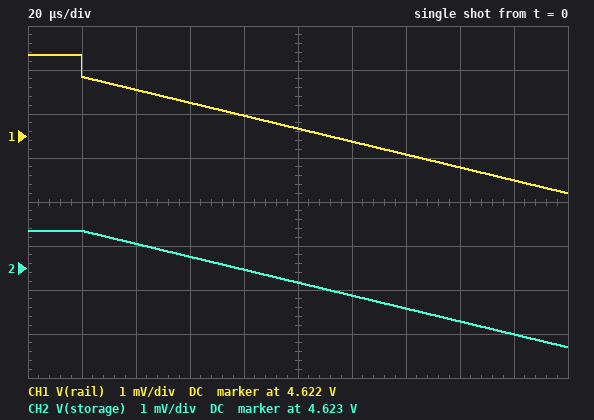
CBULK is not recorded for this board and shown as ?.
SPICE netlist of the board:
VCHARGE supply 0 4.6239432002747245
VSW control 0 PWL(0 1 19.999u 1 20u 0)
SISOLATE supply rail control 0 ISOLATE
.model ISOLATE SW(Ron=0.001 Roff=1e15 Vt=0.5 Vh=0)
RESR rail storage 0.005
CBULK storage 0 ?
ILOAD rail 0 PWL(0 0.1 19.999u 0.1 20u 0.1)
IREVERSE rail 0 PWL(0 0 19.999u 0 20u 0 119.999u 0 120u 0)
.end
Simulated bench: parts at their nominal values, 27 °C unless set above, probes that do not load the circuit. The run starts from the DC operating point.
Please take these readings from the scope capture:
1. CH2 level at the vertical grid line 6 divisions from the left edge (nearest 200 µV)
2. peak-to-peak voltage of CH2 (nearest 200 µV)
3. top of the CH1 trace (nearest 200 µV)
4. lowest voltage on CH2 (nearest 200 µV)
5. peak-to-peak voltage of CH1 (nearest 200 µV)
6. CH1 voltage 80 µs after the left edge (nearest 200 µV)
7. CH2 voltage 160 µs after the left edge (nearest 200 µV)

4.6224 V
2.6 mV
4.6238 V
4.6212 V
3.2 mV
4.6224 V
4.6218 V
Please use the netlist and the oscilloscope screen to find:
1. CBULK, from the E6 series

6.8 mF
